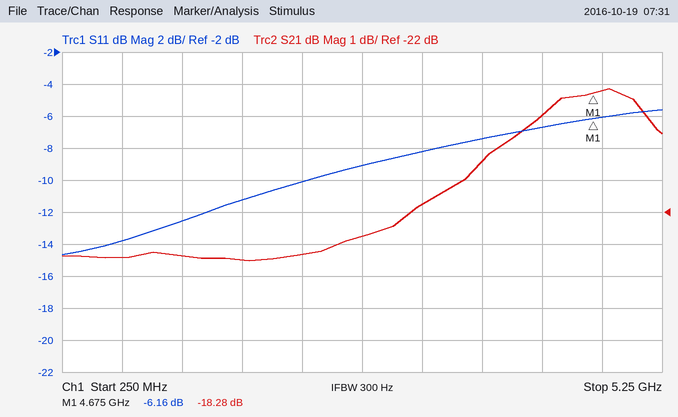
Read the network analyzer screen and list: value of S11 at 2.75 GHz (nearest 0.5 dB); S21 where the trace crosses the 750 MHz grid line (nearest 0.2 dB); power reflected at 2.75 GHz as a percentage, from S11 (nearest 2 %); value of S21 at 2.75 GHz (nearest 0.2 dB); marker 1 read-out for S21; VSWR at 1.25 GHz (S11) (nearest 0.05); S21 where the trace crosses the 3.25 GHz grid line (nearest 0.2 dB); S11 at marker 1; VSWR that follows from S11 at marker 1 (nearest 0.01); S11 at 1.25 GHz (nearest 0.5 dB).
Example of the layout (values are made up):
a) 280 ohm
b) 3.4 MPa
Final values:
a) -9.0 dB
b) -23.4 dB
c) 12 %
d) -22.8 dB
e) -18.28 dB
f) 1.60
g) -21.8 dB
h) -6.16 dB
i) 2.94
j) -12.5 dB
